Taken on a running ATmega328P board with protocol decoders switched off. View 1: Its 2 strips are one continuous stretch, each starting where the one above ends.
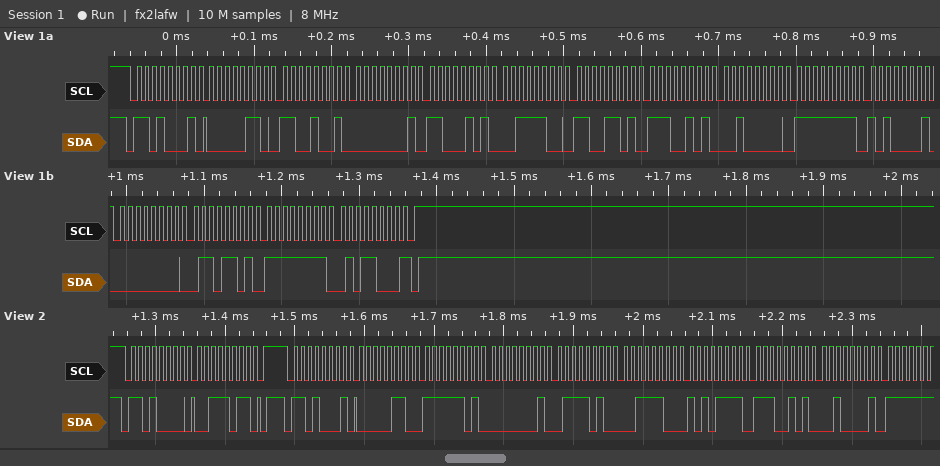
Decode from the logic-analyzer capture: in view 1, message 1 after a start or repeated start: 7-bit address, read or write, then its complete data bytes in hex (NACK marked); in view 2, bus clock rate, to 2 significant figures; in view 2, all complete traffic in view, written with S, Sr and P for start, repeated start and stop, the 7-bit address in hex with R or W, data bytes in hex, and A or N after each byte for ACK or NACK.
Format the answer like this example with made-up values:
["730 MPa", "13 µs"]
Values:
["0x68 read: 06 C9 01 C5 3C CD E5 20 FF A1 00 6D FF 58 NACK", "100 kHz", "S 68W A 3B A P S 68R A 06 A FD A 01 A 7A A 3C A AF A E5 A 21 A"]
